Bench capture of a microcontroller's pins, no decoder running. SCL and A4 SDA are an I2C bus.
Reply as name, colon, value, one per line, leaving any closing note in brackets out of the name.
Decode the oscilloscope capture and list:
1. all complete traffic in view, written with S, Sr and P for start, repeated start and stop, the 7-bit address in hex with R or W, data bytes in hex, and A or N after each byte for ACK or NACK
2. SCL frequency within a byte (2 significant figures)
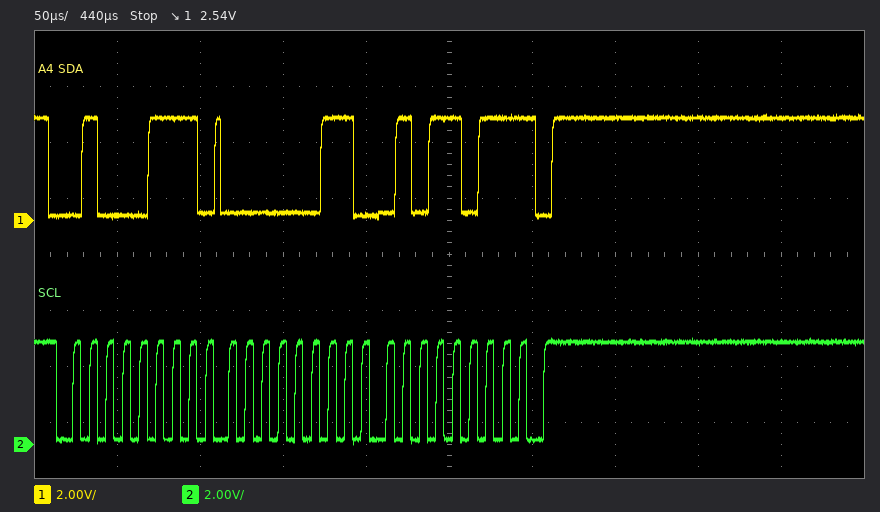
all complete traffic in view, written with S, Sr and P for start, repeated start and stop, the 7-bit address in hex with R or W, data bytes in hex, and A or N after each byte for ACK or NACK: S 23R A 03 A 5B N P
SCL frequency within a byte: 100 kHz
